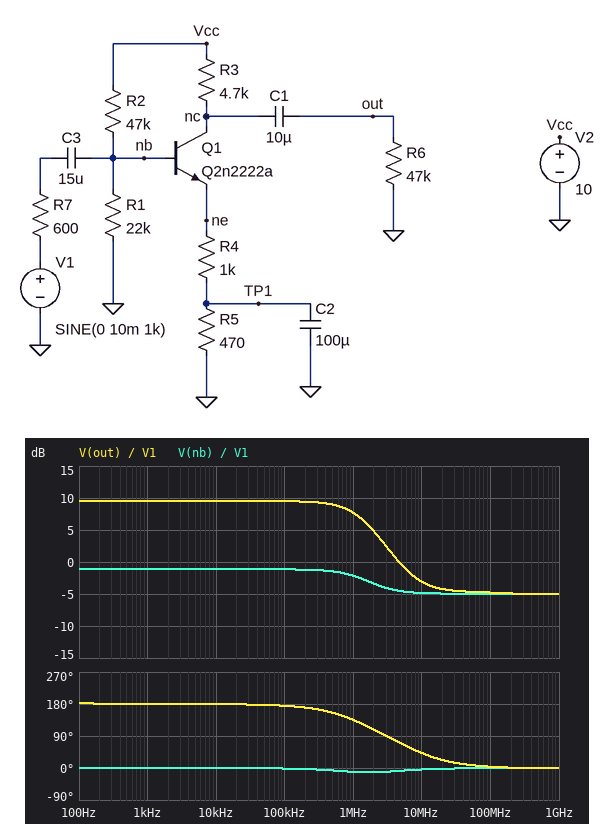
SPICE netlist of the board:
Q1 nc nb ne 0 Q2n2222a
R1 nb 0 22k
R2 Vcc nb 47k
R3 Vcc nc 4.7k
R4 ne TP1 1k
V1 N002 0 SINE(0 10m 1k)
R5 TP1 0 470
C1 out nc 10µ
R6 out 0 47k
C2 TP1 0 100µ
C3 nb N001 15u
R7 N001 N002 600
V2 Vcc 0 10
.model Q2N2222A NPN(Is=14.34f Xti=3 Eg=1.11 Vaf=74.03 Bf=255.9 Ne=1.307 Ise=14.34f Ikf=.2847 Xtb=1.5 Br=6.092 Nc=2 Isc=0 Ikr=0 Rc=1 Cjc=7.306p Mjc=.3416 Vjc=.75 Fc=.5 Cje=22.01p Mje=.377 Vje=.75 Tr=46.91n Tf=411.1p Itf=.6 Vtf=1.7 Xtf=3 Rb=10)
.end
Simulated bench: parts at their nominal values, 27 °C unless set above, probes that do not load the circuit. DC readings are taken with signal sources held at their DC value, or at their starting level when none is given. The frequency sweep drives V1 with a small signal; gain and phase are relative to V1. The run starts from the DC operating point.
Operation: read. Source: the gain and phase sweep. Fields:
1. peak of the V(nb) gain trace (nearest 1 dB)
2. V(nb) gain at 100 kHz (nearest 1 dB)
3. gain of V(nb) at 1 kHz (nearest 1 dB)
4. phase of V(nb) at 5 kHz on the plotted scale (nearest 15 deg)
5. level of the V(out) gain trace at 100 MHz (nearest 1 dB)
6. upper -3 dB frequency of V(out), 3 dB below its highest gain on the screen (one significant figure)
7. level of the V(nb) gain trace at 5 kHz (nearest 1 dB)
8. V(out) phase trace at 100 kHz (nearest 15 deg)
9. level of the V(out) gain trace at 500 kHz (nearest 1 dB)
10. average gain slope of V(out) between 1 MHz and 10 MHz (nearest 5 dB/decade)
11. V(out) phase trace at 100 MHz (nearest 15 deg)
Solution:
-1 dB
-1 dB
-1 dB
0 deg
-5 dB
1 MHz
-1 dB
180 deg
9 dB
-10 dB/decade
0 deg
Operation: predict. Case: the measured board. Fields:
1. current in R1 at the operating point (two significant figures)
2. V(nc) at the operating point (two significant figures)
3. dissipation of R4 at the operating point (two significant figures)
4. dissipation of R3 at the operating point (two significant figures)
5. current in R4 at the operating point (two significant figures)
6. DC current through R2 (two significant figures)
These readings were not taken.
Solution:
140 µA
2.5 V
2.6 mW
12 mW
1.6 mA
150 µA
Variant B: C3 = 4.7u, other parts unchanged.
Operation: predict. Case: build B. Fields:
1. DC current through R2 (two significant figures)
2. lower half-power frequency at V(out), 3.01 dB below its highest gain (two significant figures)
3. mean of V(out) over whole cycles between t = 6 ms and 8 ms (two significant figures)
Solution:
150 µA
8.5 Hz
4.2 mV
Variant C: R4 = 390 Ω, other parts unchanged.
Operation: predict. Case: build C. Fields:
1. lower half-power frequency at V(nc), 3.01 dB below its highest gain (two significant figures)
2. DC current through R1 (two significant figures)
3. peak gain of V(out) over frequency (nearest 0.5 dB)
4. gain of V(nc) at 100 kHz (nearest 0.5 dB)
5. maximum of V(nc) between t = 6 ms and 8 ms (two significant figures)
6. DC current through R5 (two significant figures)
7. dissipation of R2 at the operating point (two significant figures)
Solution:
610 kHz
100 µA
-8.5 dB
-23.5 dB
1.6 V
1.8 mA
1.3 mW
